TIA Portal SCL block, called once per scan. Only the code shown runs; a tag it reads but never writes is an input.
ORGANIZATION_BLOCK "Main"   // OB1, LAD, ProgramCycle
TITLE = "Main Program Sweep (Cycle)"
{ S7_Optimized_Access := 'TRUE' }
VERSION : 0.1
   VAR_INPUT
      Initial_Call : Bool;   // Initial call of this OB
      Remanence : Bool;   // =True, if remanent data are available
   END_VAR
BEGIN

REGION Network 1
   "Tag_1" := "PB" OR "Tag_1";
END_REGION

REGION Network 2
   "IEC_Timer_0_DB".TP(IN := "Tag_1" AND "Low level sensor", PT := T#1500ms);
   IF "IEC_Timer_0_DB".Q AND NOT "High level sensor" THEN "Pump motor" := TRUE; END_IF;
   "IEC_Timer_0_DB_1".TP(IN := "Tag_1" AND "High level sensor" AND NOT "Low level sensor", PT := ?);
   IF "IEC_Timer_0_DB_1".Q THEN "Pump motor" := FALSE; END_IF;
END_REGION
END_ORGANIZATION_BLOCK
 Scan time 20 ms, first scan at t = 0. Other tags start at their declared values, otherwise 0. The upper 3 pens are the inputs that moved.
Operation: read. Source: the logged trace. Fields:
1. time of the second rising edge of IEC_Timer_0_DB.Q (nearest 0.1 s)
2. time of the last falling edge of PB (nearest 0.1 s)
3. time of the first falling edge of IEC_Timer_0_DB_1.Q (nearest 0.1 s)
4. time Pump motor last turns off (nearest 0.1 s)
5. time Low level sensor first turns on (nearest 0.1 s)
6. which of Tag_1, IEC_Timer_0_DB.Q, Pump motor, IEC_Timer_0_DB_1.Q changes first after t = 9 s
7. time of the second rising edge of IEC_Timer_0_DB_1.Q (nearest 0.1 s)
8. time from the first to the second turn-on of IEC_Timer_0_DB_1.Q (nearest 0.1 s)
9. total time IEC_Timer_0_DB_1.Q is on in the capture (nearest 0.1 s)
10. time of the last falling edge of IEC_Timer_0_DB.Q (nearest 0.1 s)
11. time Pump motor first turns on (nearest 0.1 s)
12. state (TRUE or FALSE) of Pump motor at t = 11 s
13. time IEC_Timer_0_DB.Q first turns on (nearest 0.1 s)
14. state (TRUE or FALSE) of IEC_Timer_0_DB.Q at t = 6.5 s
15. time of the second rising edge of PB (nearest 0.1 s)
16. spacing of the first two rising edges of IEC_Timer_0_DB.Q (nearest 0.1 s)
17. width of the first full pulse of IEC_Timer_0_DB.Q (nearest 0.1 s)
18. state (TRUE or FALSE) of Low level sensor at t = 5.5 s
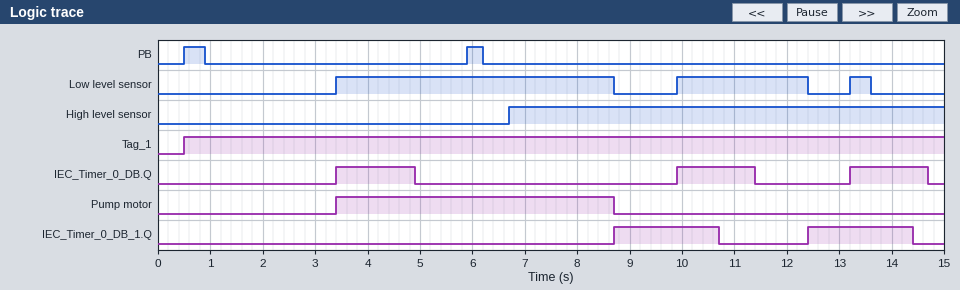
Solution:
9.9 s
6.2 s
10.7 s
8.7 s
3.4 s
IEC_Timer_0_DB.Q
12.4 s
3.7 s
4.0 s
14.7 s
3.4 s
FALSE
3.4 s
FALSE
5.9 s
6.5 s
1.5 s
TRUE
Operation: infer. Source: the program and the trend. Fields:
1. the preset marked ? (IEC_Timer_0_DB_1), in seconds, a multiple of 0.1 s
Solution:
2.0 s
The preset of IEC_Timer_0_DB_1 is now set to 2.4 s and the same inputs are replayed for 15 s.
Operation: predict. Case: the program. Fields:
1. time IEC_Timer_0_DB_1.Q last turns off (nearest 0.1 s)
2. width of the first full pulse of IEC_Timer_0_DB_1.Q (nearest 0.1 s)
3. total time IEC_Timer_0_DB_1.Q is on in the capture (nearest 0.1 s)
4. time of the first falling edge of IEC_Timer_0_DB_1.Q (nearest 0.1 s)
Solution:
14.8 s
2.4 s
4.8 s
11.1 s
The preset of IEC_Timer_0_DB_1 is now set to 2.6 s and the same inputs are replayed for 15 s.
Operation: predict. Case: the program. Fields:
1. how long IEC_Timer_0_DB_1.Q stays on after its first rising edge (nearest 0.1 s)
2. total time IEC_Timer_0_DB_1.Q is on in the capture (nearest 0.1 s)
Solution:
2.6 s
5.2 s
